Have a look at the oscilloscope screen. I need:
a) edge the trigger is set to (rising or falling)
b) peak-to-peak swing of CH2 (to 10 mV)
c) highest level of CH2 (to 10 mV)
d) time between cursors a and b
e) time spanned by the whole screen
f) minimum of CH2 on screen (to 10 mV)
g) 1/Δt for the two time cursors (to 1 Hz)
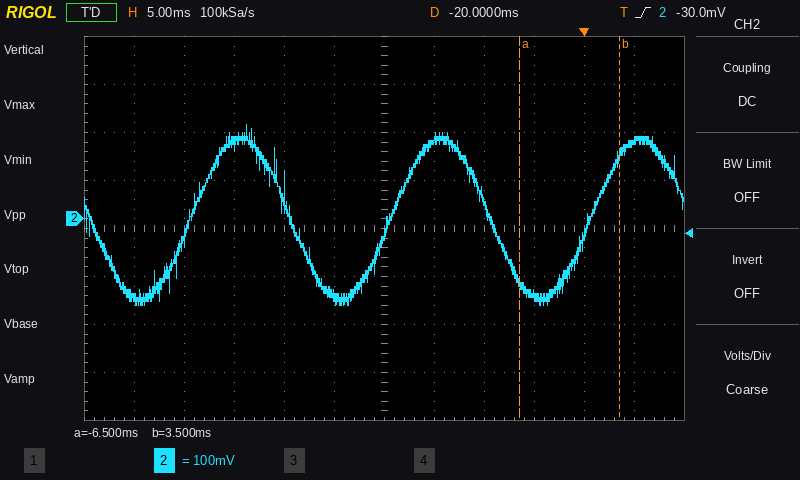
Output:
rising
380 mV
200 mV
10.0 ms
60 ms
-180 mV
100 Hz
